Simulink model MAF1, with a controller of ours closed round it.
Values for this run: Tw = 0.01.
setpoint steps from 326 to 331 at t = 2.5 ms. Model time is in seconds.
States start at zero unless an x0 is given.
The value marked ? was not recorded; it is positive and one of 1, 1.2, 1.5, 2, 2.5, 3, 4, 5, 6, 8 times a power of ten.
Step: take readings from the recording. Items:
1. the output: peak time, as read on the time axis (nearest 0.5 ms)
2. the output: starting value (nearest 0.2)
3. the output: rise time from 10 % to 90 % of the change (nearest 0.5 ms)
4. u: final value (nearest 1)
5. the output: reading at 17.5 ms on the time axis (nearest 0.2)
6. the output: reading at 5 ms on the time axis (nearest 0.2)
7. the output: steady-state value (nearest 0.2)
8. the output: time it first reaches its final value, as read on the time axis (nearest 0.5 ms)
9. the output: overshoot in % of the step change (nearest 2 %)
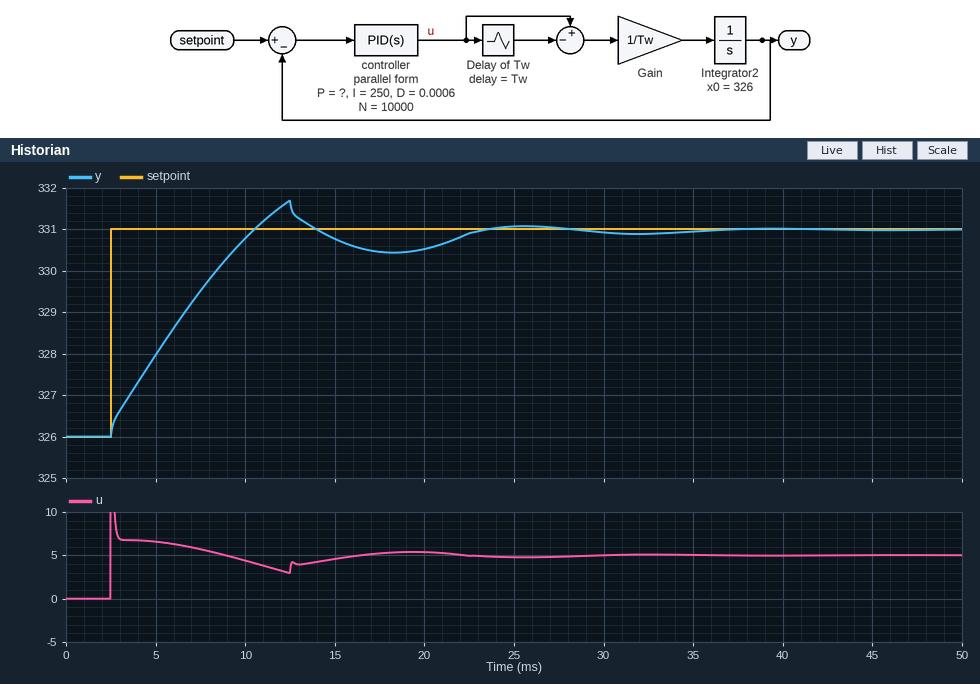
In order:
12.5 ms
326.0
6.5 ms
5
330.4
328.0
331.0
10.5 ms
14 %
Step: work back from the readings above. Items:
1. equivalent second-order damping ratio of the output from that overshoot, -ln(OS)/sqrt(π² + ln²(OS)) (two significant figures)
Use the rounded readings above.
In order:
0.53
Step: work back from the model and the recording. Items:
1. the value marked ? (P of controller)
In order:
1.5
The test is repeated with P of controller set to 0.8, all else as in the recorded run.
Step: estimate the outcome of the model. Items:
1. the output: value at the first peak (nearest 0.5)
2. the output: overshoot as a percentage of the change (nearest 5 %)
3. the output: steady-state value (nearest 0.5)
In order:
331.5
10 %
331.0
